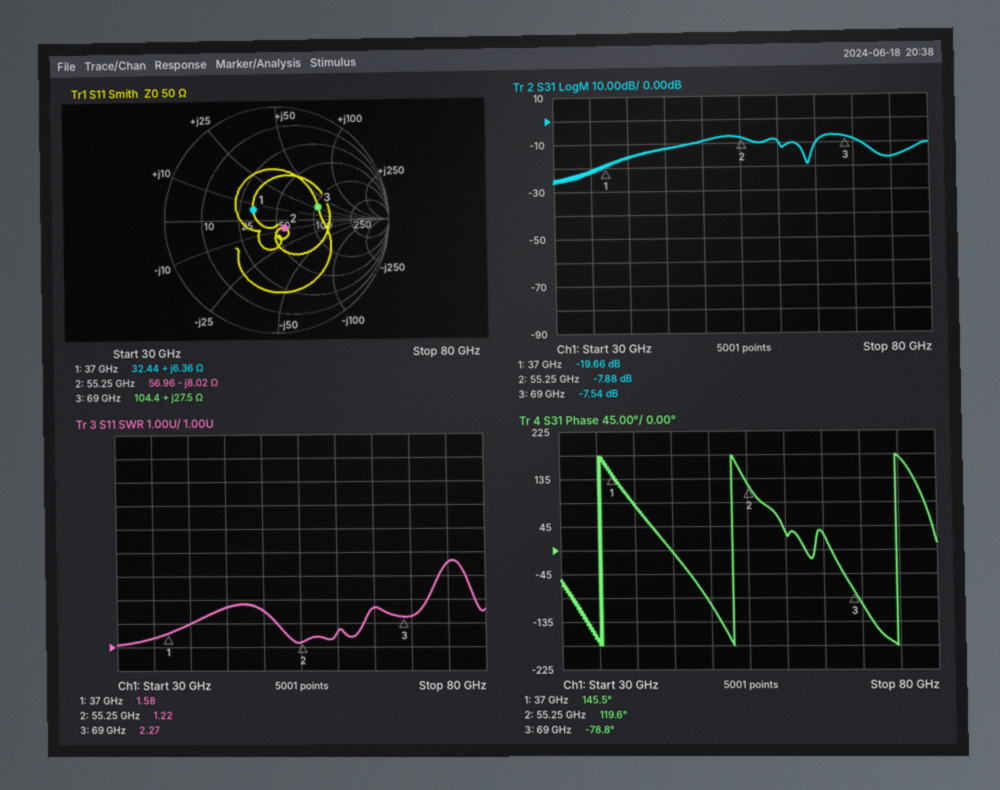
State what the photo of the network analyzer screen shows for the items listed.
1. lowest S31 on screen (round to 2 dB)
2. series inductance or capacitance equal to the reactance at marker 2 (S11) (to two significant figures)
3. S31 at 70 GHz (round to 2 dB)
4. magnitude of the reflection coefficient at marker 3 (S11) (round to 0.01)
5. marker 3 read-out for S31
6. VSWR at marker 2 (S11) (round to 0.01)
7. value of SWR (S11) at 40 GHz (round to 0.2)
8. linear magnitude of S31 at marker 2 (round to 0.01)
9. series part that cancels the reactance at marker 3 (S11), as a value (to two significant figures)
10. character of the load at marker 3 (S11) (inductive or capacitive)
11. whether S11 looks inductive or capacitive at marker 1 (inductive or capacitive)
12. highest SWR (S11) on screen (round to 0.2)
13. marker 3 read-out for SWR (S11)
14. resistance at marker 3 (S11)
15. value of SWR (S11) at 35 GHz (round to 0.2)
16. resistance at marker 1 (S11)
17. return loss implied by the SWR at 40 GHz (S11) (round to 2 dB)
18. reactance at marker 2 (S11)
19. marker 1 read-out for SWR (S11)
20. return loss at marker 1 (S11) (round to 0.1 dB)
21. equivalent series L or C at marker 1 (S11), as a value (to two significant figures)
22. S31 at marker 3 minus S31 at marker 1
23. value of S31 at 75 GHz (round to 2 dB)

-26 dB
360 fF
-8 dB
0.39
-7.54 dB
1.22
2.0
0.40
84 fF
inductive
inductive
4.6
2.27
104.4 Ω
1.4
32.44 Ω
10 dB
-8.02 Ω
1.58
12.9 dB
27 pH
12.12 dB
-16 dB
